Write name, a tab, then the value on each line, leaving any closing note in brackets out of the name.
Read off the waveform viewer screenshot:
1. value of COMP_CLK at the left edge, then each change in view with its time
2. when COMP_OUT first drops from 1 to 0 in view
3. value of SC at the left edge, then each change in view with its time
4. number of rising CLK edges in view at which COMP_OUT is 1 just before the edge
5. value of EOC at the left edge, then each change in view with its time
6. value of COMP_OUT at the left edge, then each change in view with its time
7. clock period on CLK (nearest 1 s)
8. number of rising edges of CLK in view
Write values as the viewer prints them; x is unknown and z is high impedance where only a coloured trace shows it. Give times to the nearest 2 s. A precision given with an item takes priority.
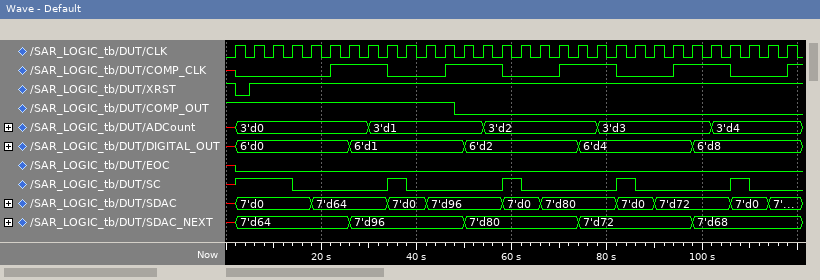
value of COMP_CLK at the left edge, then each change in view with its time	x, 0 at 2 s, 1 at 22 s, 0 at 34 s, 1 at 46 s, 0 at 58 s, 1 at 70 s, 0 at 82 s, 1 at 94 s, 0 at 106 s, 1 at 118 s
when COMP_OUT first drops from 1 to 0 in view	48 s
value of SC at the left edge, then each change in view with its time	x, 1 at 2 s, 0 at 14 s, 1 at 34 s, 0 at 38 s, 1 at 58 s, 0 at 62 s, 1 at 82 s, 0 at 86 s, 1 at 106 s, 0 at 110 s
number of rising CLK edges in view at which COMP_OUT is 1 just before the edge	12
value of EOC at the left edge, then each change in view with its time	x, 0 at 2 s
value of COMP_OUT at the left edge, then each change in view with its time	1, 0 at 48 s
clock period on CLK	4 s
number of rising edges of CLK in view	30
